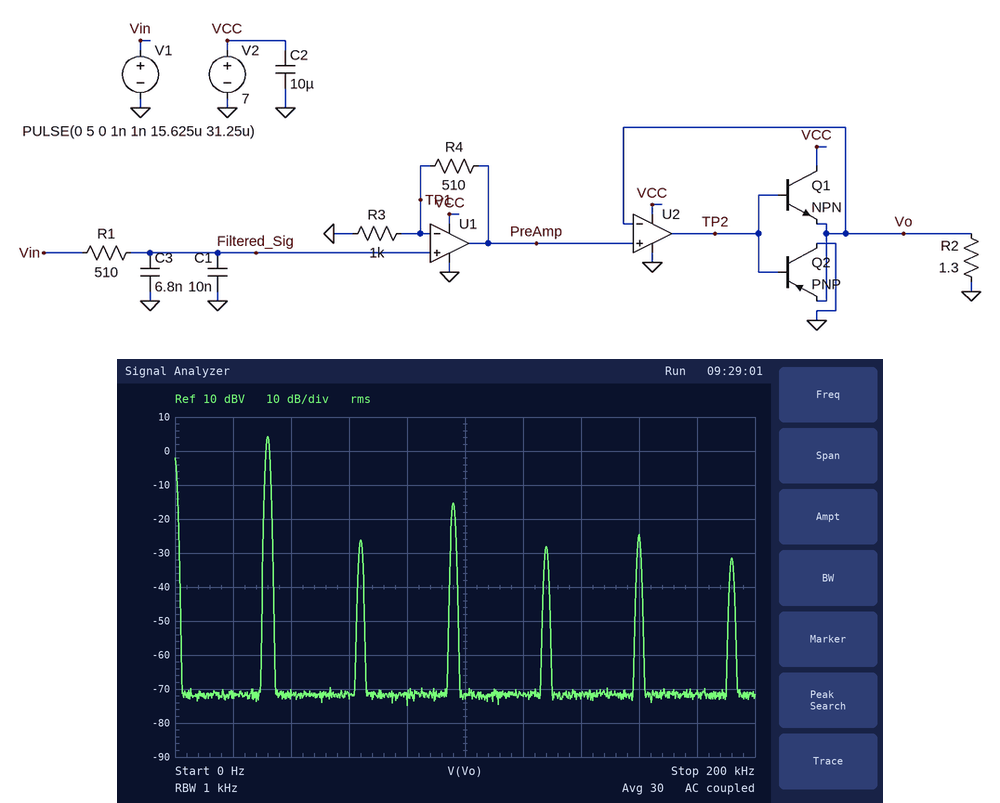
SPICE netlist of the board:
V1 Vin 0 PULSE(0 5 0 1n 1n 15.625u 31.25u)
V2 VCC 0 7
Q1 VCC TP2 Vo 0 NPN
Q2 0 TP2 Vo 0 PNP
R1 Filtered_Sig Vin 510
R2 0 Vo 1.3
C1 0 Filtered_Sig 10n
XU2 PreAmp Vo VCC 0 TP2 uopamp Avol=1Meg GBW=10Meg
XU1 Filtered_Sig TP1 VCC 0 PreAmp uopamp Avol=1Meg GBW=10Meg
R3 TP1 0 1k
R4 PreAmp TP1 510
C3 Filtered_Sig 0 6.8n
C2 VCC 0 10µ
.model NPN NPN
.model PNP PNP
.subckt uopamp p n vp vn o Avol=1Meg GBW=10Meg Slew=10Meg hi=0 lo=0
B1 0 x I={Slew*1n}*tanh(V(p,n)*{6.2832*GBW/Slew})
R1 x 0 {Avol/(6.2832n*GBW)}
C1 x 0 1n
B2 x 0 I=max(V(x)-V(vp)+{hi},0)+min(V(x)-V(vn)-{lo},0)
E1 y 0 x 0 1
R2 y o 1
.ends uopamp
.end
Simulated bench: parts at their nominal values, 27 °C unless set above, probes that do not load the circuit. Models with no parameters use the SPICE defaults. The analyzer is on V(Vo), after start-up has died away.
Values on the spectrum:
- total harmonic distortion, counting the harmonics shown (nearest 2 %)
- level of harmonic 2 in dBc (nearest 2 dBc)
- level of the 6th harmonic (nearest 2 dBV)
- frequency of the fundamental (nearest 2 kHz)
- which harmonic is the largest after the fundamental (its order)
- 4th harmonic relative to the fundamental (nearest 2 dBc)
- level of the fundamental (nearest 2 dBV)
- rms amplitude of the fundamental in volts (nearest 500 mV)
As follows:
12 %
-30 dBc
-32 dBV
32 kHz
3
-32 dBc
4 dBV
1.5 V
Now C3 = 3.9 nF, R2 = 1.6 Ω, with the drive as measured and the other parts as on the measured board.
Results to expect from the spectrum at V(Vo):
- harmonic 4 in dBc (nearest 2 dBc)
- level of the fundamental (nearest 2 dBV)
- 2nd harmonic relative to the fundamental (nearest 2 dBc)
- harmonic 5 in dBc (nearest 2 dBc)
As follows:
-30 dBc
6 dBV
-24 dBc
-26 dBc
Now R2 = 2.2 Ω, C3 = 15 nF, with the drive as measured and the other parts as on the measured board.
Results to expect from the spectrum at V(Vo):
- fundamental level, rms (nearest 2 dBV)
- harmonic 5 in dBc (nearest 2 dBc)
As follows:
2 dBV
-28 dBc
